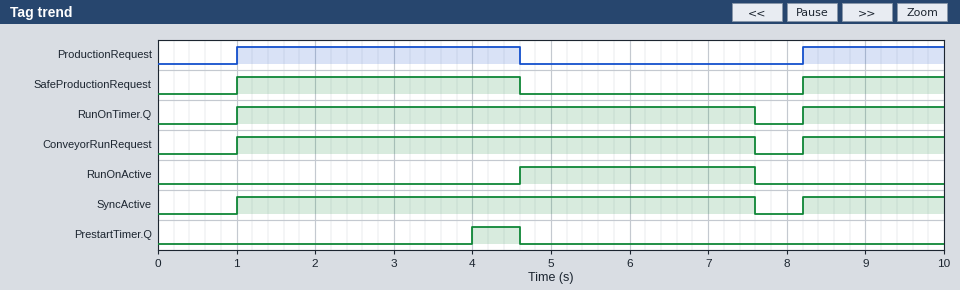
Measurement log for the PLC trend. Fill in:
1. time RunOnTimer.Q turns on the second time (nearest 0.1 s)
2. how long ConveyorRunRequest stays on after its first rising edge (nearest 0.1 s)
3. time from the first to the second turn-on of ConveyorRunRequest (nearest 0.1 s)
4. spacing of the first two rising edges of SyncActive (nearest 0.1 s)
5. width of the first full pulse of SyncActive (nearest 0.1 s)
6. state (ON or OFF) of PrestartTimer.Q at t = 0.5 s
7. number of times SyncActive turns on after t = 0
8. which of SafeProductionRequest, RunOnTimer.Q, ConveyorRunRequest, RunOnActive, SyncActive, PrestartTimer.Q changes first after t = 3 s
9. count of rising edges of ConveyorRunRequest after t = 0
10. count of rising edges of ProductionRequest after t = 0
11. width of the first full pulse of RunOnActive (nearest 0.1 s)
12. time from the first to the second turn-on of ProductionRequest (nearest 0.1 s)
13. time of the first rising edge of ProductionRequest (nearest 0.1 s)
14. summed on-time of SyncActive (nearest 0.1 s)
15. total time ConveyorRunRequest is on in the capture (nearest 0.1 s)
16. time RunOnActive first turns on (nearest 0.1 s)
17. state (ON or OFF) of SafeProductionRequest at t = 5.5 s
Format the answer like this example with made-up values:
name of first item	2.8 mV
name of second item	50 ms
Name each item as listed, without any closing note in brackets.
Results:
time RunOnTimer.Q turns on the second time	8.2 s
how long ConveyorRunRequest stays on after its first rising edge	6.6 s
time from the first to the second turn-on of ConveyorRunRequest	7.2 s
spacing of the first two rising edges of SyncActive	7.2 s
width of the first full pulse of SyncActive	6.6 s
state (ON or OFF) of PrestartTimer.Q at t = 0.5 s	OFF
number of times SyncActive turns on after t = 0	2
which of SafeProductionRequest, RunOnTimer.Q, ConveyorRunRequest, RunOnActive, SyncActive, PrestartTimer.Q changes first after t = 3 s	PrestartTimer.Q
count of rising edges of ConveyorRunRequest after t = 0	2
count of rising edges of ProductionRequest after t = 0	2
width of the first full pulse of RunOnActive	3.0 s
time from the first to the second turn-on of ProductionRequest	7.2 s
time of the first rising edge of ProductionRequest	1.0 s
summed on-time of SyncActive	8.4 s
total time ConveyorRunRequest is on in the capture	8.4 s
time RunOnActive first turns on	4.6 s
state (ON or OFF) of SafeProductionRequest at t = 5.5 s	OFF
